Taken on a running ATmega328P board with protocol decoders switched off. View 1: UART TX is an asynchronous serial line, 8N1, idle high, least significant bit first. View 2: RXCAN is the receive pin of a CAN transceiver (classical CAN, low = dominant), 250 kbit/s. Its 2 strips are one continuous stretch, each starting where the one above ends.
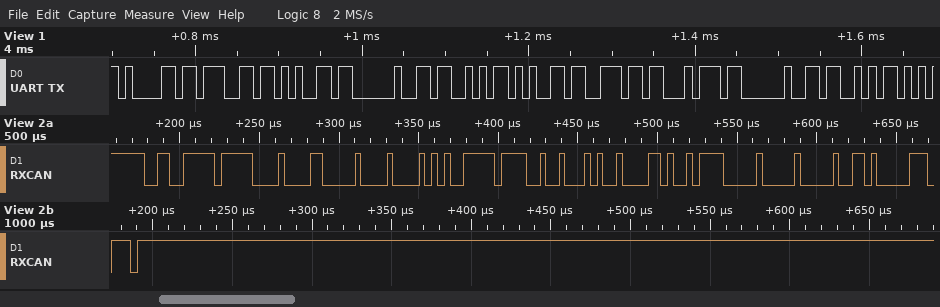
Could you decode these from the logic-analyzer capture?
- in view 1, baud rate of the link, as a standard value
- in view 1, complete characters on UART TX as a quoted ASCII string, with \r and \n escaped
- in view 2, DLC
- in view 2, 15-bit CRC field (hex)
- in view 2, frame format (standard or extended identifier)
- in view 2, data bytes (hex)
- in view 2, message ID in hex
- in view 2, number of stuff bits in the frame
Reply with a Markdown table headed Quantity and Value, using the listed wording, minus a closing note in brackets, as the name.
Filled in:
| Quantity | Value |
|---|---|
| in view 1, baud rate of the link, as a standard value | 115200 baud |
| in view 1, complete characters on UART TX as a quoted ASCII string, with \r and \n escaped | "age Sent S" |
| in view 2, DLC | 8 |
| in view 2, 15-bit CRC field | 0x341B |
| in view 2, frame format | extended |
| in view 2, data bytes | 54 FF 92 29 0D 2F 00 00 |
| in view 2, message ID in hex | 0x0CFF10C0 |
| in view 2, number of stuff bits in the frame | 8 |
